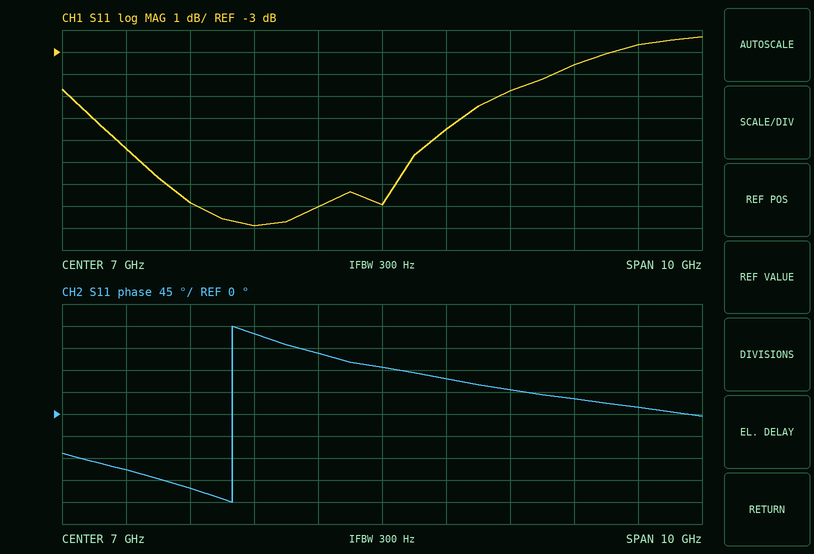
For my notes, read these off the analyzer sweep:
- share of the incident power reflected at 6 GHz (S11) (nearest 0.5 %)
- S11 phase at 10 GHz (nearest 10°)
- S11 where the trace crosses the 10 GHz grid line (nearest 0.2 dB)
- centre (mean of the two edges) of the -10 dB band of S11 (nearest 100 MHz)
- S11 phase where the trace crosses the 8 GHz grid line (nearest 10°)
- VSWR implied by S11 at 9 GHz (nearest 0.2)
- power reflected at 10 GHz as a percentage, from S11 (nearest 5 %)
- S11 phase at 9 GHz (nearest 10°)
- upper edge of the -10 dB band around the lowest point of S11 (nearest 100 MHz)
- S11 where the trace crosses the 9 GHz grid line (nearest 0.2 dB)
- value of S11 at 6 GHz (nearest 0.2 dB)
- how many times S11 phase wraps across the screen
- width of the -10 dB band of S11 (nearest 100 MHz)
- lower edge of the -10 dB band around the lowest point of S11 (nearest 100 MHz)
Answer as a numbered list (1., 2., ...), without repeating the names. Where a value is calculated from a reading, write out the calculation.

1. 10^(-10/10) ≈ 10.0 %
2. 30°
3. -3.6 dB
4. 5.1 GHz
5. 70°
6. |Γ| = 10^(-4.8/20) = 0.5754; VSWR = (1 + 0.5754)/(1 − 0.5754) ≈ 3.71, so 3.8 to the nearest 0.2
7. 10^(-3.6/10) ≈ 43.7 %, so 45 % to the nearest 5 %
8. 50°
9. 6.0 GHz
10. -4.8 dB
11. -10.0 dB
12. 1
13. 6.0 GHz − 4.1 GHz = 1.9 GHz
14. 4.1 GHz
